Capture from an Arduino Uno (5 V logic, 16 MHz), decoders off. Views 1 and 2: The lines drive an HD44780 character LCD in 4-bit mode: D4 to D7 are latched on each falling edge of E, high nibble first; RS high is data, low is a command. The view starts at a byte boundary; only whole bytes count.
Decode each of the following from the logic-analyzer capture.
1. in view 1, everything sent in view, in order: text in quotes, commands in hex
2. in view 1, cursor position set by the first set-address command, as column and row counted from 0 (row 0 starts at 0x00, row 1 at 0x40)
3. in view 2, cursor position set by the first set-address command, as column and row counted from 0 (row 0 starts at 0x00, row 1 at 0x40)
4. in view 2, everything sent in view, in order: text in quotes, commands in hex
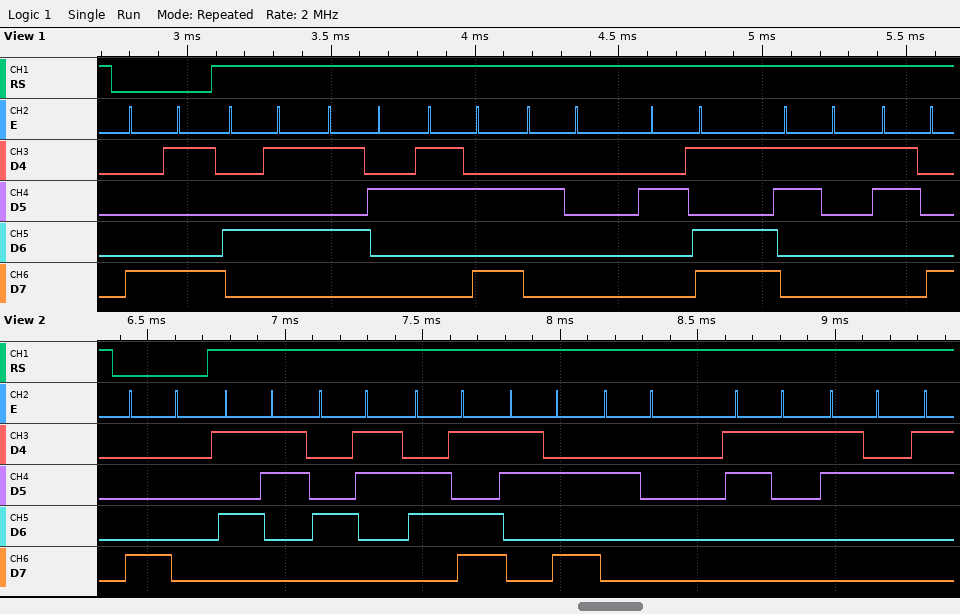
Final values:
0x89 "ER: -18"
column 9, row 0
column 0, row 0
0x80 "SCm: 12"
